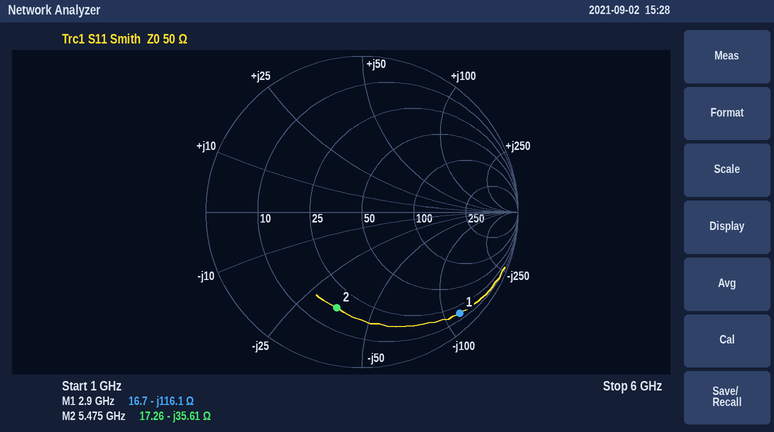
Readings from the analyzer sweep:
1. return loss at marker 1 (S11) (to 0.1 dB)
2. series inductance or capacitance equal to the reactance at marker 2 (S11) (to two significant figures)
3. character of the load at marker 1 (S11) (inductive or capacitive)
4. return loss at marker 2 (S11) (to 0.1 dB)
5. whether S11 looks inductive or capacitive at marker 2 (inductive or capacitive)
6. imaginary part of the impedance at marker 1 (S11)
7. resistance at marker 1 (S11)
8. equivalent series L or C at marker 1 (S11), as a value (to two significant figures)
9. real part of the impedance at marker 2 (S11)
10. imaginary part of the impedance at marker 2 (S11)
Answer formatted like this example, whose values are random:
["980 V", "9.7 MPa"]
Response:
["0.9 dB", "820 fF", "capacitive", "3.9 dB", "capacitive", "-116.1 Ω", "16.7 Ω", "470 fF", "17.26 Ω", "-35.61 Ω"]
